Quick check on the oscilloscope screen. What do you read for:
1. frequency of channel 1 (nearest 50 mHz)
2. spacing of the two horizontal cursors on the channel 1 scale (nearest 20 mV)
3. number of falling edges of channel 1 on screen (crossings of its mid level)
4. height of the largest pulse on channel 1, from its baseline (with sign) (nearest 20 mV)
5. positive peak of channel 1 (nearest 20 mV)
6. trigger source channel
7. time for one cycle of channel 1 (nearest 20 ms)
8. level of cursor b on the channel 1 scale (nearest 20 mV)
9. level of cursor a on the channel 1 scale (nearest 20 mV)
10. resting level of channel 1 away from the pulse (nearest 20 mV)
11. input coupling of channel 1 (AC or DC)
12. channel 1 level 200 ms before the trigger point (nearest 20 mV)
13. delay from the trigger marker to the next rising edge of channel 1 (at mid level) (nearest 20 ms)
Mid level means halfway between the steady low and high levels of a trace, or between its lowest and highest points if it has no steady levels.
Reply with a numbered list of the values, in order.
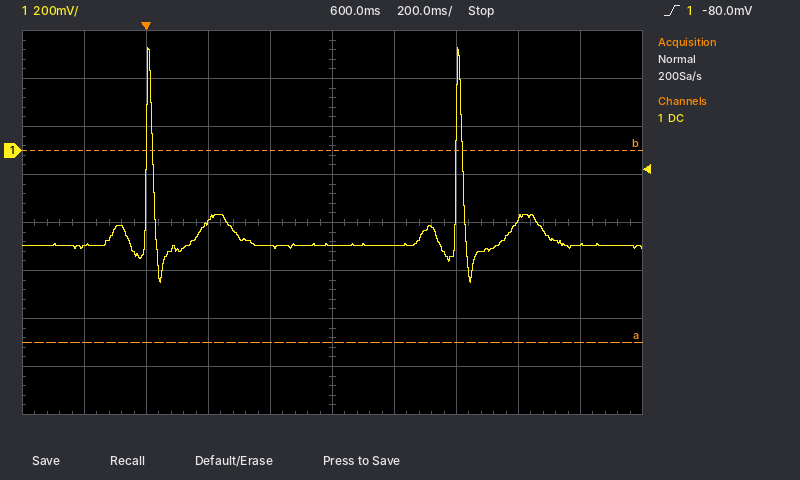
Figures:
1. 1.00 Hz
2. 800 mV
3. 2
4. +820 mV
5. 420 mV
6. channel 1
7. 1.00 s
8. 0 mV
9. -800 mV
10. -400 mV
11. DC
12. -400 mV
13. 1.00 s
